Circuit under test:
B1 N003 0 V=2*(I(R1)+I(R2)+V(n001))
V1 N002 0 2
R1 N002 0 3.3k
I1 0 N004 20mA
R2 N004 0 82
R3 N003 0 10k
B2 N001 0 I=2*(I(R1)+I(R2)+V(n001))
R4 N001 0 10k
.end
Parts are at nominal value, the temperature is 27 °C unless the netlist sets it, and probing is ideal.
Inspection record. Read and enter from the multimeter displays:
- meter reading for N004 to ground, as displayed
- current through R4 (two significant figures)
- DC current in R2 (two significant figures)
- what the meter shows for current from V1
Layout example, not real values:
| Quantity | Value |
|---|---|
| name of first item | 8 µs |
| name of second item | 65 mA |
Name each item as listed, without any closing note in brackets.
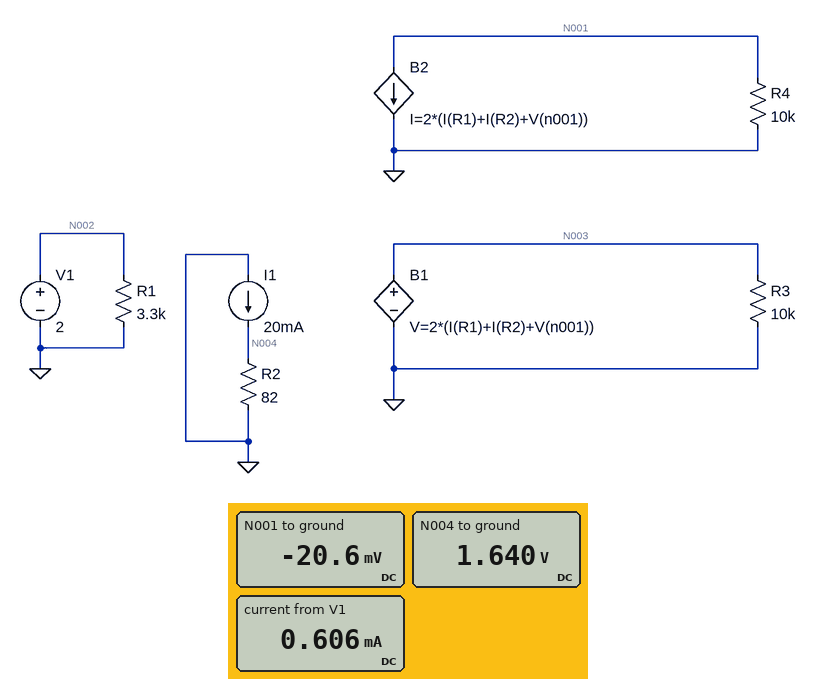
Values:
| Quantity | Value |
|---|---|
| meter reading for N004 to ground, as displayed | 1.640 V |
| current through R4 | 2.1 µA |
| DC current in R2 | 20 mA |
| what the meter shows for current from V1 | 0.606 mA |
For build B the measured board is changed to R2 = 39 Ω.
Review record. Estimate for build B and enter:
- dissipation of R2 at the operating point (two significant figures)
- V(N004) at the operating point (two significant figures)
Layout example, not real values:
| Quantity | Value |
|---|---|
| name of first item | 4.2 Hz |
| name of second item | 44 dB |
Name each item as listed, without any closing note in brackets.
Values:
| Quantity | Value |
|---|---|
| dissipation of R2 at the operating point | 16 mW |
| V(N004) at the operating point | 780 mV |
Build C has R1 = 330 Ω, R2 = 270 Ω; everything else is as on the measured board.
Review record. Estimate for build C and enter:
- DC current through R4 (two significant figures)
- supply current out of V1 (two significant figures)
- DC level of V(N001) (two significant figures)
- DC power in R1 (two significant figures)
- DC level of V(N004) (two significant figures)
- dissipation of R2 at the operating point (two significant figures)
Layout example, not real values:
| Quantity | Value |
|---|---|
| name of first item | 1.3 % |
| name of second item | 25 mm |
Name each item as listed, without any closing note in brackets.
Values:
| Quantity | Value |
|---|---|
| DC current through R4 | 2.6 µA |
| supply current out of V1 | 6.1 mA |
| DC level of V(N001) | -26 mV |
| DC power in R1 | 12 mW |
| DC level of V(N004) | 5.4 V |
| dissipation of R2 at the operating point | 110 mW |
